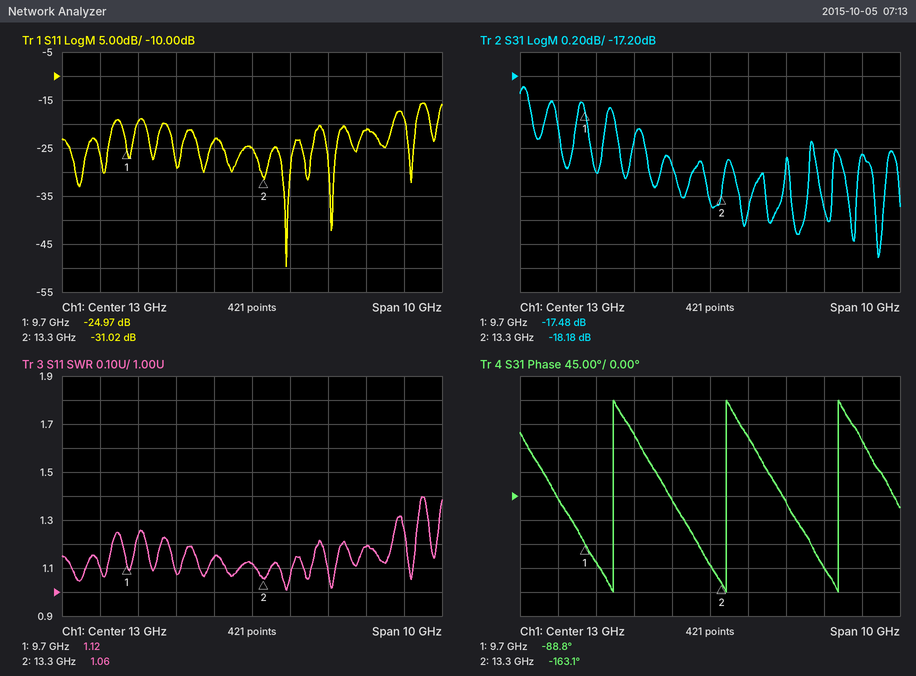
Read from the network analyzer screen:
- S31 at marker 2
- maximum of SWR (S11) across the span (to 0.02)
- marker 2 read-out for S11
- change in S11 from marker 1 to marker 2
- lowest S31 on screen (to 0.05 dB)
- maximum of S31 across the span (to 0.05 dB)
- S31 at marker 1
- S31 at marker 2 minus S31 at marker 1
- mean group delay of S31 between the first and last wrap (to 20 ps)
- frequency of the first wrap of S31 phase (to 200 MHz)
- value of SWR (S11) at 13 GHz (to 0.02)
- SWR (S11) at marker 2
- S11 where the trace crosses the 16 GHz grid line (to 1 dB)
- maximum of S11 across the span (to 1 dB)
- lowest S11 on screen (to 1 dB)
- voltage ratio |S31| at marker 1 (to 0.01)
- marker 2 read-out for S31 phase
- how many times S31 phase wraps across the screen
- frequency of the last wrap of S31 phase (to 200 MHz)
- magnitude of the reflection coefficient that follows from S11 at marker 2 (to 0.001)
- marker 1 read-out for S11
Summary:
-18.18 dB
1.40
-31.02 dB
-6.05 dB
-18.70 dB
-17.30 dB
-17.48 dB
-0.70 dB
340 ps
10.4 GHz
1.12
1.06
-21 dB
-16 dB
-50 dB
0.13
-163.1°
3
16.4 GHz
0.028
-24.97 dB
